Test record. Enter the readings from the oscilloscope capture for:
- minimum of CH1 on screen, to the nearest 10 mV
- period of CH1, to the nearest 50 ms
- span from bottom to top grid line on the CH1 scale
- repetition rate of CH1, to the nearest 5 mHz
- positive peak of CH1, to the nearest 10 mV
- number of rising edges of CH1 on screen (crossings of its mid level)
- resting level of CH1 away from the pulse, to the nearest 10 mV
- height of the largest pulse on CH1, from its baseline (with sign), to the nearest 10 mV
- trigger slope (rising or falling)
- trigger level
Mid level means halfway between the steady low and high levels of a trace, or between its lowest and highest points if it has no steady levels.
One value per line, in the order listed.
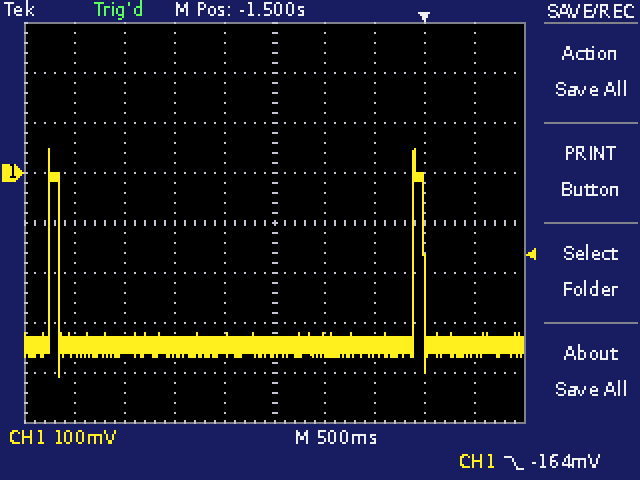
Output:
-410 mV
3.65 s
800 mV
275 mHz
50 mV
2
-340 mV
+390 mV
falling
-164 mV
